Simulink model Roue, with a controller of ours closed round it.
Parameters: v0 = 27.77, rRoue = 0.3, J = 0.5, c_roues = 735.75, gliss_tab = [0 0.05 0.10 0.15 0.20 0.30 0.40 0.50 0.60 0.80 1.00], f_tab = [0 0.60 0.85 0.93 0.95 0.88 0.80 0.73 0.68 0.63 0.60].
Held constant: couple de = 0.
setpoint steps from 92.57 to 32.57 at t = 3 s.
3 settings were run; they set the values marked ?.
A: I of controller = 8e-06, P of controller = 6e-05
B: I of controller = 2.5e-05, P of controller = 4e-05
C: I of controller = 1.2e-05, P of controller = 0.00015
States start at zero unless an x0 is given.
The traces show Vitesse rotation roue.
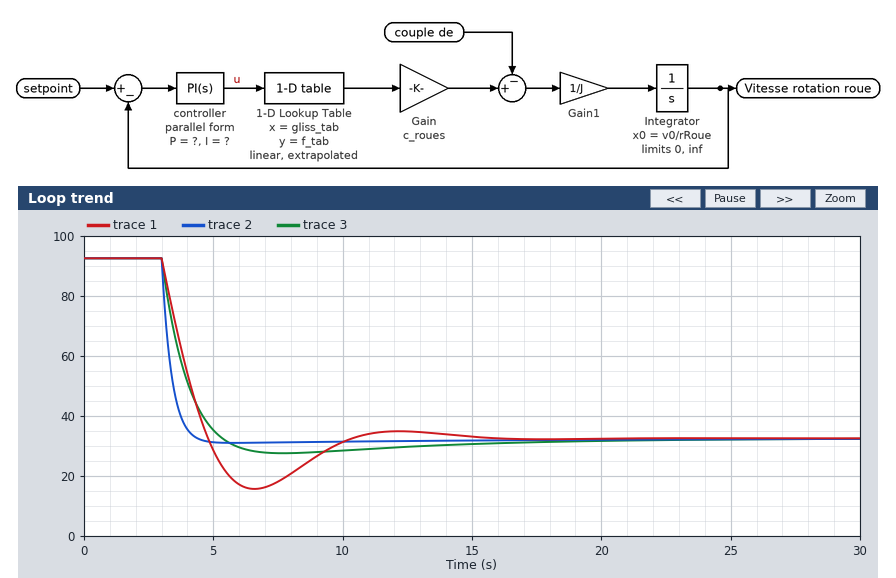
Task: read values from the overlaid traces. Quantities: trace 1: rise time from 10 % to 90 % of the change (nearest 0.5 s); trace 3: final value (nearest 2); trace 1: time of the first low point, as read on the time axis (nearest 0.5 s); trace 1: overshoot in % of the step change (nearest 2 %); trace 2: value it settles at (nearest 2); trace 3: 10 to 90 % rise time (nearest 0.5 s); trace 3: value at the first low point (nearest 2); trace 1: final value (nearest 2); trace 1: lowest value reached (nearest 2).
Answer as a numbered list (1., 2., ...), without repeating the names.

1. 1.5 s
2. 32
3. 6.5 s
4. 28 %
5. 32
6. 1.5 s
7. 28
8. 32
9. 16
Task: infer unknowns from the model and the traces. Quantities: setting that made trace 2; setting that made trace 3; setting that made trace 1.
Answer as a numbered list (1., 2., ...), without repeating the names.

1. C
2. A
3. B
